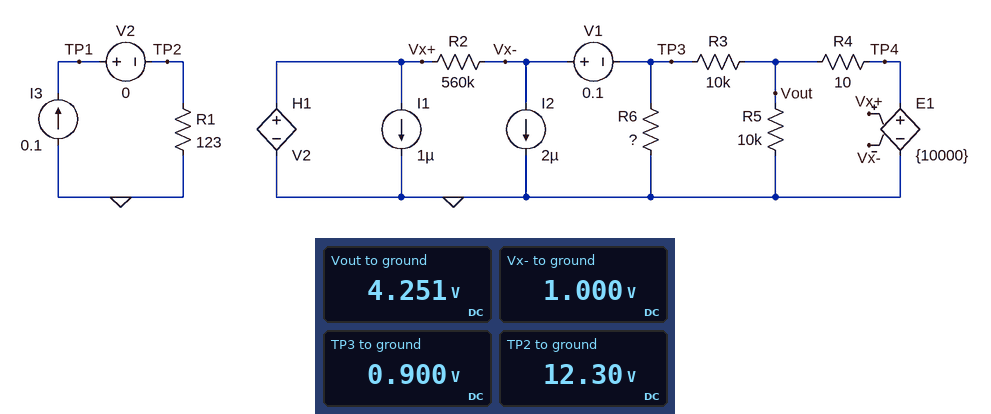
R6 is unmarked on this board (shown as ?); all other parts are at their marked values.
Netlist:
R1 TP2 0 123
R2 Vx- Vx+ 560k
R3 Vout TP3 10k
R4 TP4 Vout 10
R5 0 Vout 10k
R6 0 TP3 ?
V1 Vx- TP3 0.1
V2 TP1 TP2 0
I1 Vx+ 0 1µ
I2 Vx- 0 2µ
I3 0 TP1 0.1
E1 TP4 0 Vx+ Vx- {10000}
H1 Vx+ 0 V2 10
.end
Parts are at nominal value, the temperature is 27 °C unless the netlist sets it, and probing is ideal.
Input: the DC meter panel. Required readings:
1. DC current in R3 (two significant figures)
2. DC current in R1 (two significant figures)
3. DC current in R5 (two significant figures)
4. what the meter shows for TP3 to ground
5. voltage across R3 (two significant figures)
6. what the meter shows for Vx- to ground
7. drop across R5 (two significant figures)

340 µA
100 mA
430 µA
0.900 V
3.4 V
1.000 V
4.3 V
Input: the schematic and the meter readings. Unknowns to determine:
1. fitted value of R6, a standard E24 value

2.7 kΩ
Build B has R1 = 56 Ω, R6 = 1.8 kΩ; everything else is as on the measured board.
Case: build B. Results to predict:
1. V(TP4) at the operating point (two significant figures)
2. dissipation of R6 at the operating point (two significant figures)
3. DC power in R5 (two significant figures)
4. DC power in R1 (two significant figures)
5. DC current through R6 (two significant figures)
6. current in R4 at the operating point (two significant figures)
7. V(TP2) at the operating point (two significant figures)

5.9 V
450 µW
3.5 mW
560 mW
500 µA
1.1 mA
5.6 V
